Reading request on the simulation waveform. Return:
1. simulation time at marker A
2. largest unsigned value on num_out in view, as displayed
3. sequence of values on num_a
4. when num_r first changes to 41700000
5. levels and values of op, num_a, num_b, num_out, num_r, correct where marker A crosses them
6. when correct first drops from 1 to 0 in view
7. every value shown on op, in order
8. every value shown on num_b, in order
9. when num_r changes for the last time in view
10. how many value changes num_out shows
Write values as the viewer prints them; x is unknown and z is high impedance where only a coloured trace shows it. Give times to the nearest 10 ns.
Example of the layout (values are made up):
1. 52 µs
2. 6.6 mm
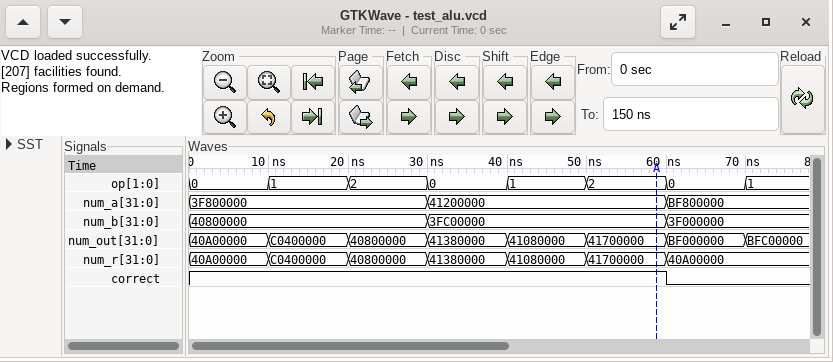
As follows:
1. 60 ns
2. C0400000
3. 3F800000, 41200000, BF800000
4. 50 ns
5. op=2, num_a=41200000, num_b=3FC00000, num_out=41700000, num_r=41700000, correct=1
6. 60 ns
7. 0, 1, 2, 0, 1, 2, 0, 1
8. 40800000, 3FC00000, 3F000000
9. 60 ns
10. 7
